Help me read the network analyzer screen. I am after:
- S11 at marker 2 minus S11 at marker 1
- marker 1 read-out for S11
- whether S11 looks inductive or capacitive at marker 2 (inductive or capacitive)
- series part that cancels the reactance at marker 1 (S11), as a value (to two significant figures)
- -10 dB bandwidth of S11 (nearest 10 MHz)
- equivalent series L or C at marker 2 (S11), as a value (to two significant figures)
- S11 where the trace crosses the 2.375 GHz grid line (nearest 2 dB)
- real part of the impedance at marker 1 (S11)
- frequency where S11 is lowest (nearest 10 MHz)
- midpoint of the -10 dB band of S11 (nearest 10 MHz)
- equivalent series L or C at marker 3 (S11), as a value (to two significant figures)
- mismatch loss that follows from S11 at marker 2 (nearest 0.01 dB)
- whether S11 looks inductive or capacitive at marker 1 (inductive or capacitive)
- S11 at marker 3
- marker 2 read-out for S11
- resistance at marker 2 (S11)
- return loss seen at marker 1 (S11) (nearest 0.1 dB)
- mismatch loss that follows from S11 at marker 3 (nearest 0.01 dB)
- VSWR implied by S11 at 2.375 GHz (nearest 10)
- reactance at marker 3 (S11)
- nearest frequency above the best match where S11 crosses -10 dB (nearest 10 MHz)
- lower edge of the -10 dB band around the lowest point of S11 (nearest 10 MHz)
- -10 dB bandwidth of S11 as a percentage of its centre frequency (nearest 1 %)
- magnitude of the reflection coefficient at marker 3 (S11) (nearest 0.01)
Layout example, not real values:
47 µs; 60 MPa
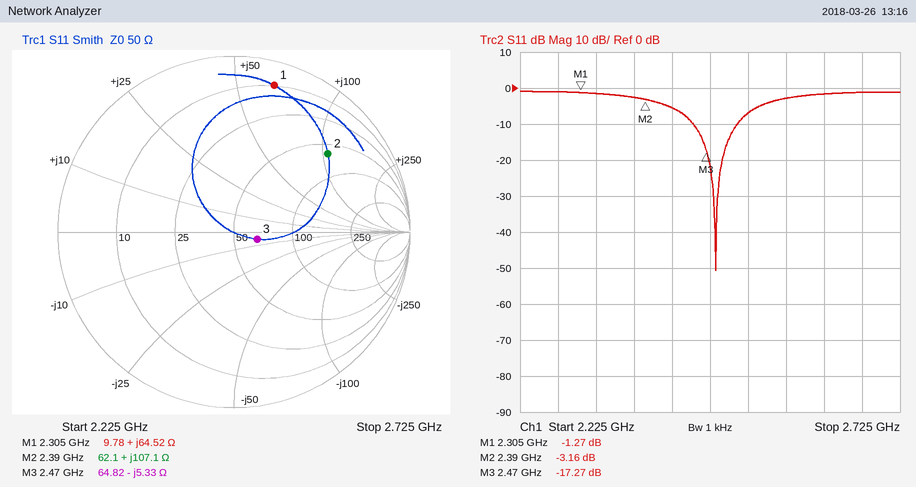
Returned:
-1.89 dB; -1.27 dB; inductive; 1.1 pF; 60 MHz; 7.1 nH; -2 dB; 9.78 Ω; 2.48 GHz; 2.48 GHz; 12 pF; 2.87 dB; inductive; -17.27 dB; -3.16 dB; 62.1 Ω; 1.3 dB; 0.08 dB; 10; -5.33 Ω; 2.51 GHz; 2.45 GHz; 2 %; 0.14
